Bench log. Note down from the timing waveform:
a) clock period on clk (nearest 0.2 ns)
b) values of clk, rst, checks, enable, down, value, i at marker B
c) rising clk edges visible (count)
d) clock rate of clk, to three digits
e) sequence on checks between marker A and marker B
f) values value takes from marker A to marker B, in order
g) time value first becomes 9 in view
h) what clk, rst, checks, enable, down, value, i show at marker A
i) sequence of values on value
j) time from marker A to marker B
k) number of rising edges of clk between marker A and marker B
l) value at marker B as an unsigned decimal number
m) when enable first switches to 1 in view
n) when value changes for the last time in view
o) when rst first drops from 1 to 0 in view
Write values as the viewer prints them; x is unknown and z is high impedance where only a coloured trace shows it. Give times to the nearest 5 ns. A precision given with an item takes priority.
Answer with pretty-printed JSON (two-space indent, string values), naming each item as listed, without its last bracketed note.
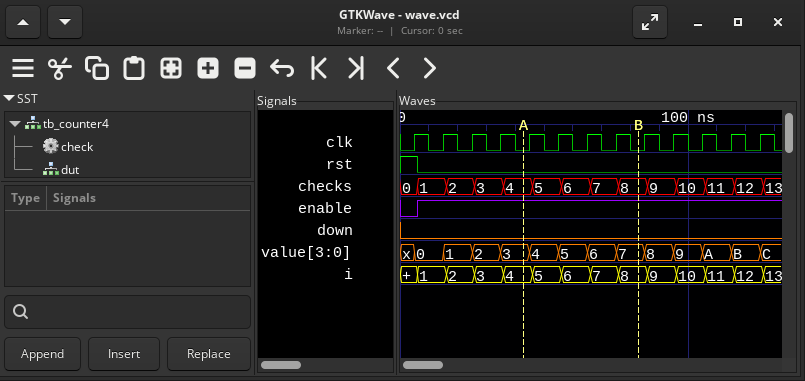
{
  "clock period on clk": "10 ns",
  "values of clk, rst, checks, enable, down, value, i at marker B": "clk=0, rst=0, checks=8, enable=1, down=0, value=7, i=8",
  "rising clk edges visible": "13",
  "clock rate of clk, to three digits": "100 MHz",
  "sequence on checks between marker A and marker B": "4, 5, 6, 7, 8",
  "values value takes from marker A to marker B, in order": "3, 4, 5, 6, 7",
  "time value first becomes 9 in view": "95 ns",
  "what clk, rst, checks, enable, down, value, i show at marker A": "clk=0, rst=0, checks=4, enable=1, down=0, value=3, i=4",
  "sequence of values on value": "x, 0, 1, 2, 3, 4, 5, 6, 7, 8, 9, A, B, C",
  "time from marker A to marker B": "40 ns",
  "number of rising edges of clk between marker A and marker B": "4",
  "value at marker B as an unsigned decimal number": "7",
  "when enable first switches to 1 in view": "5 ns",
  "when value changes for the last time in view": "125 ns",
  "when rst first drops from 1 to 0 in view": "5 ns"
}
